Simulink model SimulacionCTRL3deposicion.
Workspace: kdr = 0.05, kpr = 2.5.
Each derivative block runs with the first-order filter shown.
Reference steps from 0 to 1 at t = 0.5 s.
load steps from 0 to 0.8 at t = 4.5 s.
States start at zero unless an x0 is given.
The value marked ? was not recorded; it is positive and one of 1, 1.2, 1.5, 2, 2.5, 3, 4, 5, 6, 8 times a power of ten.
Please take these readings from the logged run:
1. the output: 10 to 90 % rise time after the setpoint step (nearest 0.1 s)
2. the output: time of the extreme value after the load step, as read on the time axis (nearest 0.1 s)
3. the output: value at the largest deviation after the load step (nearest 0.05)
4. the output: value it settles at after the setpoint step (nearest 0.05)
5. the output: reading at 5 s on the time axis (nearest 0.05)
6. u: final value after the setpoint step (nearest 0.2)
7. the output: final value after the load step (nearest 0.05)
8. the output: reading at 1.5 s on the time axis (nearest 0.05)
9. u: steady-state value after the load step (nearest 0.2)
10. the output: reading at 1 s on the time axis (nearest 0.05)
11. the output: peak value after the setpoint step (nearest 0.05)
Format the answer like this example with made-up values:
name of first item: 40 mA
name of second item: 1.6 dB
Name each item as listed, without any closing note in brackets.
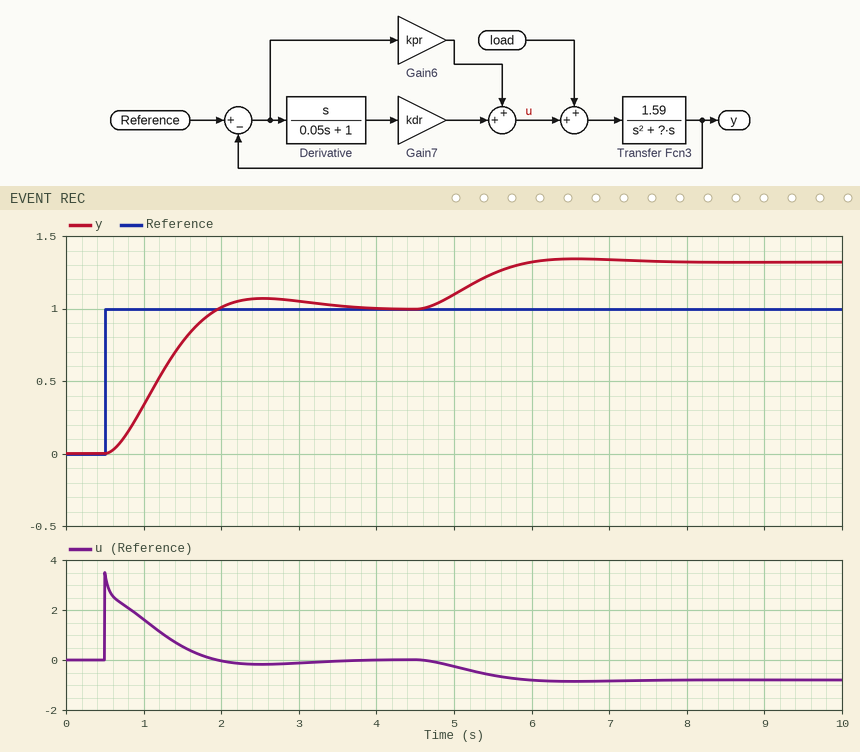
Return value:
the output: 10 to 90 % rise time after the setpoint step: 1.0 s
the output: time of the extreme value after the load step, as read on the time axis: 6.6 s
the output: value at the largest deviation after the load step: 1.35
the output: value it settles at after the setpoint step: 1.00
the output: reading at 5 s on the time axis: 1.10
u: final value after the setpoint step: 0.0
the output: final value after the load step: 1.30
the output: reading at 1.5 s on the time axis: 0.75
u: steady-state value after the load step: -0.8
the output: reading at 1 s on the time axis: 0.35
the output: peak value after the setpoint step: 1.05
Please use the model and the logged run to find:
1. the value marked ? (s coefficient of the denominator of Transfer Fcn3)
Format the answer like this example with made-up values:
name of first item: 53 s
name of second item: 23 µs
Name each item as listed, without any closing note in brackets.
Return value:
the value marked ?: 2.5
